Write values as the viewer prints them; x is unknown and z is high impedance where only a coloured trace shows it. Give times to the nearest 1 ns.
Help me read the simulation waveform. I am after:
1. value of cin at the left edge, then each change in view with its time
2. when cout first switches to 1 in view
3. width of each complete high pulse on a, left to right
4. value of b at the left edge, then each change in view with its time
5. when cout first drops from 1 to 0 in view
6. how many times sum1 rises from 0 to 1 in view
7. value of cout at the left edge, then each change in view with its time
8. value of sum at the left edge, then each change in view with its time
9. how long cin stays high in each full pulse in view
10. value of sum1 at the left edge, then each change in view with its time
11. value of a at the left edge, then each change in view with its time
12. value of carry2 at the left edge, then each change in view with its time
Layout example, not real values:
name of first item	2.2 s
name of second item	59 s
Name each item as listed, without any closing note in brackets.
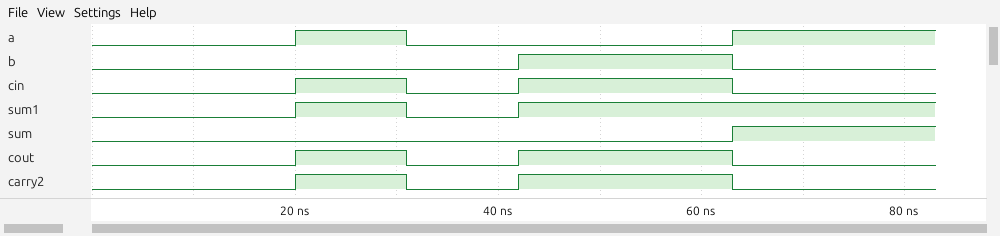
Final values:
value of cin at the left edge, then each change in view with its time	0, 1 at 20 ns, 0 at 31 ns, 1 at 42 ns, 0 at 63 ns
when cout first switches to 1 in view	20 ns
width of each complete high pulse on a, left to right	11 ns
value of b at the left edge, then each change in view with its time	0, 1 at 42 ns, 0 at 63 ns
when cout first drops from 1 to 0 in view	31 ns
how many times sum1 rises from 0 to 1 in view	2
value of cout at the left edge, then each change in view with its time	0, 1 at 20 ns, 0 at 31 ns, 1 at 42 ns, 0 at 63 ns
value of sum at the left edge, then each change in view with its time	0, 1 at 63 ns
how long cin stays high in each full pulse in view	11 ns, 21 ns
value of sum1 at the left edge, then each change in view with its time	0, 1 at 20 ns, 0 at 31 ns, 1 at 42 ns
value of a at the left edge, then each change in view with its time	0, 1 at 20 ns, 0 at 31 ns, 1 at 63 ns
value of carry2 at the left edge, then each change in view with its time	0, 1 at 20 ns, 0 at 31 ns, 1 at 42 ns, 0 at 63 ns
